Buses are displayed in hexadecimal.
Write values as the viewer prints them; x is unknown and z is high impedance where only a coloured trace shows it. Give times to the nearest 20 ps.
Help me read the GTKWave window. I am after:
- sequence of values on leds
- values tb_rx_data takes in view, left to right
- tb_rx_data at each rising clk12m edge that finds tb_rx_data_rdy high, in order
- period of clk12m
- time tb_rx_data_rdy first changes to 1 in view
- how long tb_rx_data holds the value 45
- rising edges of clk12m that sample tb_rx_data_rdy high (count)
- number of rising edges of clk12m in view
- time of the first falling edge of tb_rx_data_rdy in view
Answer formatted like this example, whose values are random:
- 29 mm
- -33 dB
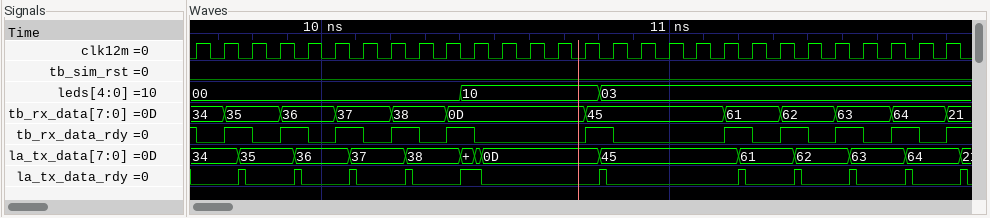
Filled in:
- 00, 10, 03
- 34, 35, 36, 37, 38, 0D, 45, 61, 62, 63, 64, 21
- 34, 35, 36, 37, 38, 0D, 45, 61, 62, 63, 64
- 80 ps
- 9720 ps
- 400 ps
- 11
- 28
- 9640 ps
